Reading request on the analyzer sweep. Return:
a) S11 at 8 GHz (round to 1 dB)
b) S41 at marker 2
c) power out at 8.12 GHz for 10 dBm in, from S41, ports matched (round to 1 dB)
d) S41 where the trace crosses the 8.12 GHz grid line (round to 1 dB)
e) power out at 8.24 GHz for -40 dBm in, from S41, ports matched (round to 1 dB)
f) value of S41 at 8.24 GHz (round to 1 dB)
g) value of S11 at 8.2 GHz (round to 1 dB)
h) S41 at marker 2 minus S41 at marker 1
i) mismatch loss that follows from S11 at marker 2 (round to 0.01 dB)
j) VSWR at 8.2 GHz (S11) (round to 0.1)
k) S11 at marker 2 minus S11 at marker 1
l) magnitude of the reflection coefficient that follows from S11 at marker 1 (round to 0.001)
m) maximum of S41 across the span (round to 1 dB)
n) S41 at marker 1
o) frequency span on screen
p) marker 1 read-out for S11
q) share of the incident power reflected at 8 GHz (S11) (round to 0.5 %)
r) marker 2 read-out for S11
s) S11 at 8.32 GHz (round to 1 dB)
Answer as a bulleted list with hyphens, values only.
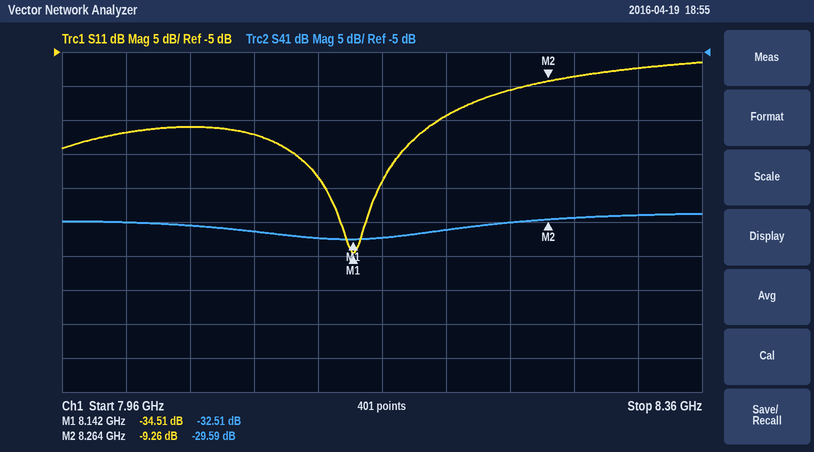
- -17 dB
- -29.59 dB
- -22 dBm
- -32 dB
- -70 dBm
- -30 dB
- -14 dB
- 2.92 dB
- 0.55 dB
- 1.5
- 25.25 dB
- 0.019
- -29 dB
- -32.51 dB
- 400 MHz
- -34.51 dB
- 2.0 %
- -9.26 dB
- -7 dB
